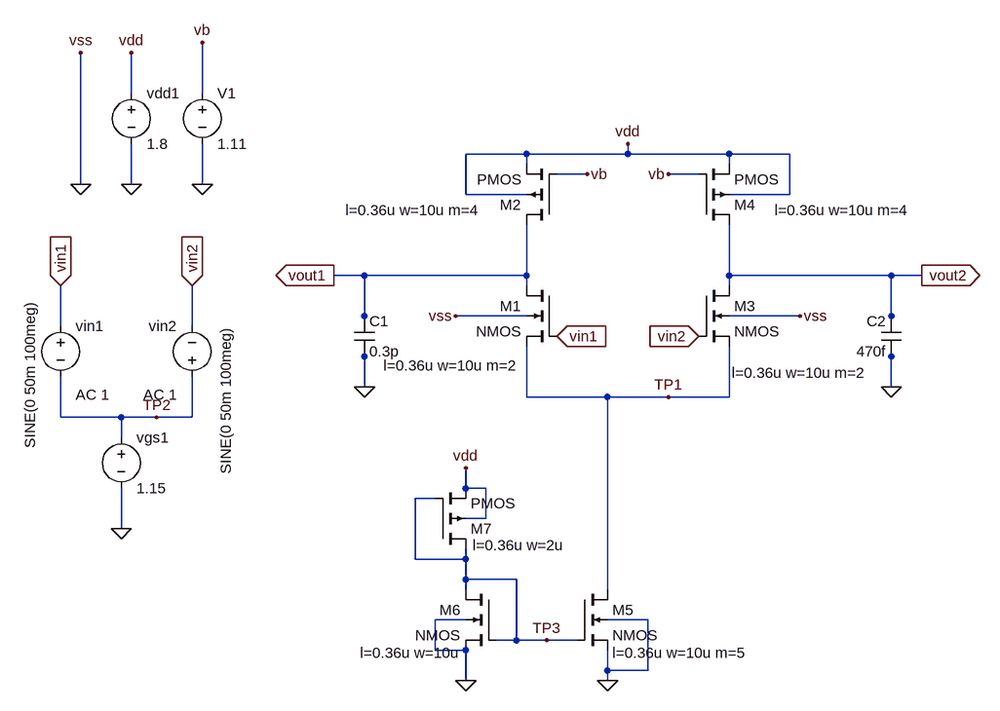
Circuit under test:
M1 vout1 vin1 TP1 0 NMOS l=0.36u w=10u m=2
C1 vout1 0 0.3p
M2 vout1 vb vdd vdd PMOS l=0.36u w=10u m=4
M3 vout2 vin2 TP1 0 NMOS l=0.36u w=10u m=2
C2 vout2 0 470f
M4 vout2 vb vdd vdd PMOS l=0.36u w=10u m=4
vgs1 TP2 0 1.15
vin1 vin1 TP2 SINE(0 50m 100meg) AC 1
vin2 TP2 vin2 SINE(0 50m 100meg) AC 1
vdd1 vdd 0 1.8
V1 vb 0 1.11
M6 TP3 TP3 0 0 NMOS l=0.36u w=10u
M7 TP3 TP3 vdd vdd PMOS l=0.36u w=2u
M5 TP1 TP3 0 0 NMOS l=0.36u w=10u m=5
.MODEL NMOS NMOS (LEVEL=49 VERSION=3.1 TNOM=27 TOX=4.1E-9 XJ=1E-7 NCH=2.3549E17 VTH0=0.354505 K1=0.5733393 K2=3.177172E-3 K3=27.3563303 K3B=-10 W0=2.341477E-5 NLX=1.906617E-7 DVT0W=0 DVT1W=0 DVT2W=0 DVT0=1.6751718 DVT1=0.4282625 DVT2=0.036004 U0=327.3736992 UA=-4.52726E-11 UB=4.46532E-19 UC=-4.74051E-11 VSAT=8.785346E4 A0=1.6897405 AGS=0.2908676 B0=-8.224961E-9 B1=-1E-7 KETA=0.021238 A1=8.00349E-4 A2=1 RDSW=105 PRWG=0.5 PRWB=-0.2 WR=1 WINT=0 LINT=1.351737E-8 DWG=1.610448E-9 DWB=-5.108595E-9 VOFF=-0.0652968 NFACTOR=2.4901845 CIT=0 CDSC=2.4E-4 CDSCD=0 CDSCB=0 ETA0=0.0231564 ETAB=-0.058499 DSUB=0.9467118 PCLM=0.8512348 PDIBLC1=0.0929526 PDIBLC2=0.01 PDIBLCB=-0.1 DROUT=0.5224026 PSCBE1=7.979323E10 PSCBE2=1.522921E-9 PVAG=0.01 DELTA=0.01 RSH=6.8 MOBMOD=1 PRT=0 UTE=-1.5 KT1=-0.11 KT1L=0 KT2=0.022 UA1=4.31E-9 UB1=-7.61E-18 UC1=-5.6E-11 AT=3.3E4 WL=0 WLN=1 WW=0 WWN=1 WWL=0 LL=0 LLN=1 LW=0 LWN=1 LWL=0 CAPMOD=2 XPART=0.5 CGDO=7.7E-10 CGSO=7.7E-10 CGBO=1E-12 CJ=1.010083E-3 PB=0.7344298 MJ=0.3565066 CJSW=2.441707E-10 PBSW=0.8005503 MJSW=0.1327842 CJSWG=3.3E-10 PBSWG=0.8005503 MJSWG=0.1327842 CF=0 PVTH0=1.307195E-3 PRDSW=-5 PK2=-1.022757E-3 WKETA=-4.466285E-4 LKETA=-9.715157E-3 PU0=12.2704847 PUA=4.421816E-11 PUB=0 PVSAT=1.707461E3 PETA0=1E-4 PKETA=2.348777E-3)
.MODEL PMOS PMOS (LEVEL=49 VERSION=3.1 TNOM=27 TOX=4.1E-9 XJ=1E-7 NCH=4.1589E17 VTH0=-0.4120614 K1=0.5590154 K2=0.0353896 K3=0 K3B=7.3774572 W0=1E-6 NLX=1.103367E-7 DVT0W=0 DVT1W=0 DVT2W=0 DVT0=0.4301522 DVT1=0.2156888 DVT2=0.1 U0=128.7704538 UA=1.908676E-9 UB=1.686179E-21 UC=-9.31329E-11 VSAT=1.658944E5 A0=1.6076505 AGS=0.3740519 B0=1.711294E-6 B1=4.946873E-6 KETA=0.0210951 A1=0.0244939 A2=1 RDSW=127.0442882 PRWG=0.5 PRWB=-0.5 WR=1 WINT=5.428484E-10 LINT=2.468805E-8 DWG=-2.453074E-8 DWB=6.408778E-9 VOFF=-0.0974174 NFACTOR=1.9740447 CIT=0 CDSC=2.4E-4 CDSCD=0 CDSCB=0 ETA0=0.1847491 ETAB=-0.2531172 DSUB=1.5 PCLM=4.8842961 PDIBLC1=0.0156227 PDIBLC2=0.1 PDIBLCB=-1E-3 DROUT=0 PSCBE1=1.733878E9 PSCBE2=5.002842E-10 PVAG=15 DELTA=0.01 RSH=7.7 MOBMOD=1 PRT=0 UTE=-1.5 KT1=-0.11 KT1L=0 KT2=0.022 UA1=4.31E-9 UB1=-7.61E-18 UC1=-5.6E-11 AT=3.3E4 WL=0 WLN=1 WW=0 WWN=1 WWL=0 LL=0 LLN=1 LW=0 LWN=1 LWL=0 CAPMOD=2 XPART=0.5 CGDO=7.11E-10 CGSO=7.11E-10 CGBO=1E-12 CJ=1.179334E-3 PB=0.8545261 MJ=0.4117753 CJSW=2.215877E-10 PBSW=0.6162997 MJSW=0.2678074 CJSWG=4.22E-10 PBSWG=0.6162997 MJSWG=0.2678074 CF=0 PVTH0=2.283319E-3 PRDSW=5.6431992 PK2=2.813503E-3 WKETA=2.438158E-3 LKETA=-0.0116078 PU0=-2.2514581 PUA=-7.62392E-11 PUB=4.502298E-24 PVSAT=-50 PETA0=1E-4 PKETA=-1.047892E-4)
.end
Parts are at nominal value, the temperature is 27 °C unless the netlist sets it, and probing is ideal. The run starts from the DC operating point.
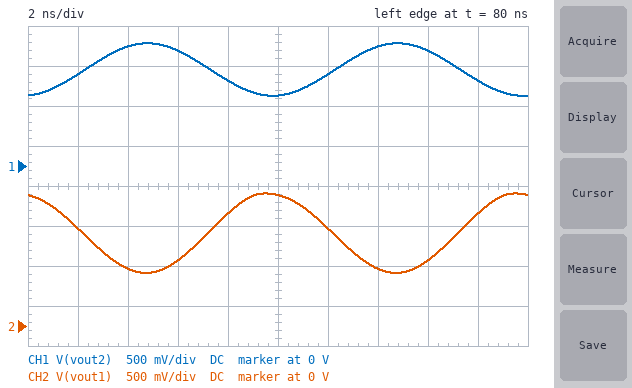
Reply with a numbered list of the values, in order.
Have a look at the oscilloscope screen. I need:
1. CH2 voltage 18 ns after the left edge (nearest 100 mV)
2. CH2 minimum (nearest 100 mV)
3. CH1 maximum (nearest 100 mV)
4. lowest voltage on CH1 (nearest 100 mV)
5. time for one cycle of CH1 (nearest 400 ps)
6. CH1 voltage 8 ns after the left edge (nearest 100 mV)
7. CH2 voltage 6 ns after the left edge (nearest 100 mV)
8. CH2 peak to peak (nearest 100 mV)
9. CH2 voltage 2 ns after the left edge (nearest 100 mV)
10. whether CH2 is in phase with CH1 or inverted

1. 1.4 V
2. 700 mV
3. 1.5 V
4. 900 mV
5. 10.0 ns
6. 1.1 V
7. 800 mV
8. 1.0 V
9. 1.2 V
10. inverted
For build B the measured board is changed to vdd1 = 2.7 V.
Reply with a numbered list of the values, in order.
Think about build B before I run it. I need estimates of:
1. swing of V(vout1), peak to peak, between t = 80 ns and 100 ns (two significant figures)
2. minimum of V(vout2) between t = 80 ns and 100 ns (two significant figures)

1. 58 mV
2. 2.6 V
